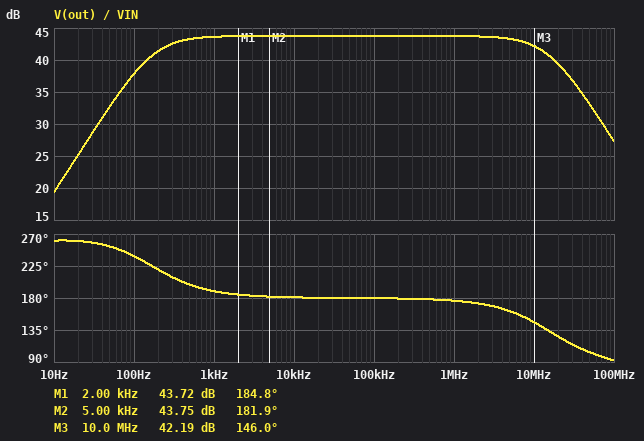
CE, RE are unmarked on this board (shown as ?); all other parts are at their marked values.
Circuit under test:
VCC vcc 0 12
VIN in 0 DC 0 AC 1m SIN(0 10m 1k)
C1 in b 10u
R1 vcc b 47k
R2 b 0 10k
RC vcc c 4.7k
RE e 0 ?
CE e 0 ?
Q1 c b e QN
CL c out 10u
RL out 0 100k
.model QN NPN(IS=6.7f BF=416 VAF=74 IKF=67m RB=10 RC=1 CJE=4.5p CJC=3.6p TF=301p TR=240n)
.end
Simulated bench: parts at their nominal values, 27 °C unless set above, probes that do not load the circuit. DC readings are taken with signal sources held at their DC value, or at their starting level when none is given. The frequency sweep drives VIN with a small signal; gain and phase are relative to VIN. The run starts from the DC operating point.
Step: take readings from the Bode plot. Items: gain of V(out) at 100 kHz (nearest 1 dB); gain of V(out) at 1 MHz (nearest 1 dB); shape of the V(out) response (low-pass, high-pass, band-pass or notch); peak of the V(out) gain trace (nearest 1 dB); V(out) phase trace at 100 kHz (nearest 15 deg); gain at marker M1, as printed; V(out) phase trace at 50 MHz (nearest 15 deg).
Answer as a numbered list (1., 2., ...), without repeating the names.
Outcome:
1. 44 dB
2. 44 dB
3. band-pass
4. 44 dB
5. 180 deg
6. 43.72 dB
7. 105 deg
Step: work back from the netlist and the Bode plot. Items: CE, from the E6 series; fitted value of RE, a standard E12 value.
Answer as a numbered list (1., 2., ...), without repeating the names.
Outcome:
1. 33 µF
2. 1.5 kΩ
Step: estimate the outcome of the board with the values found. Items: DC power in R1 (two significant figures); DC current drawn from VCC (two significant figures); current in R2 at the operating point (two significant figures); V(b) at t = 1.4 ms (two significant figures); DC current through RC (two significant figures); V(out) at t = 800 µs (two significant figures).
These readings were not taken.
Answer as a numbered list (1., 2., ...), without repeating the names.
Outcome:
1. 2.1 mW
2. 1.2 mA
3. 210 µA
4. 2.1 V
5. 950 µA
6. 1.3 V
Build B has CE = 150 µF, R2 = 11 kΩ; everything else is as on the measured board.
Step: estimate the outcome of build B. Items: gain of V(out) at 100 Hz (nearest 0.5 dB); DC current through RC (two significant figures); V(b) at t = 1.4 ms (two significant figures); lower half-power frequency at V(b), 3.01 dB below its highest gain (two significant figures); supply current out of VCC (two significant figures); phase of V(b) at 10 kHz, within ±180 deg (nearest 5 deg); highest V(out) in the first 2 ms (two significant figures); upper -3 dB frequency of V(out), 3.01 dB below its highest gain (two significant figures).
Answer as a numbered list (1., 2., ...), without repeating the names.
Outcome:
1. 44.0 dB
2. 1.1 mA
3. 2.3 V
4. 1.9 Hz
5. 1.3 mA
6. 0 deg
7. 1.5 V
8. 14 MHz
